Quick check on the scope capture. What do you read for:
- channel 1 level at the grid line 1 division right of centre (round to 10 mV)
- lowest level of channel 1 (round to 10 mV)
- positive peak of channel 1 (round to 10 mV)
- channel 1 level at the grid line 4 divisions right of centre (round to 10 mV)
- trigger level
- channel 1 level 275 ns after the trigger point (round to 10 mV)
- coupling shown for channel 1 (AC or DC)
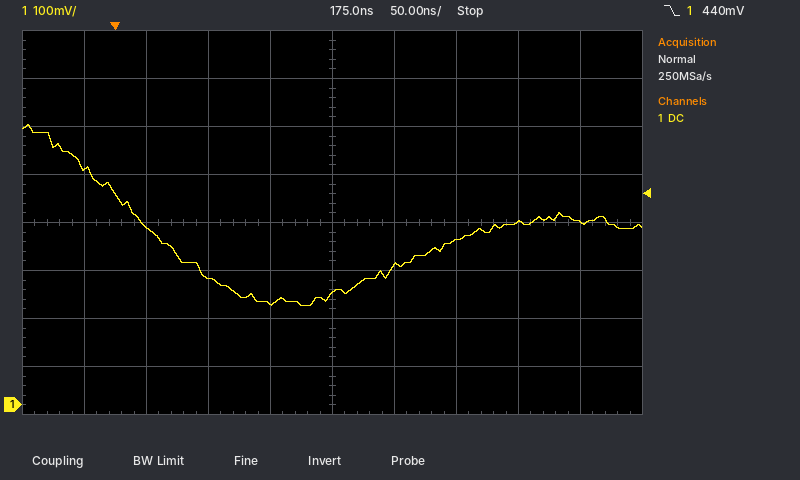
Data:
290 mV
210 mV
580 mV
380 mV
440 mV
340 mV
DC
